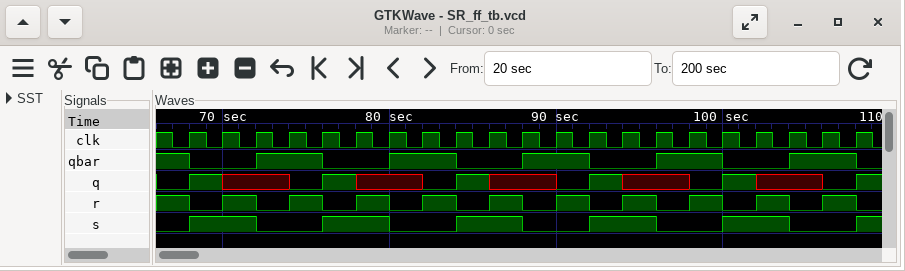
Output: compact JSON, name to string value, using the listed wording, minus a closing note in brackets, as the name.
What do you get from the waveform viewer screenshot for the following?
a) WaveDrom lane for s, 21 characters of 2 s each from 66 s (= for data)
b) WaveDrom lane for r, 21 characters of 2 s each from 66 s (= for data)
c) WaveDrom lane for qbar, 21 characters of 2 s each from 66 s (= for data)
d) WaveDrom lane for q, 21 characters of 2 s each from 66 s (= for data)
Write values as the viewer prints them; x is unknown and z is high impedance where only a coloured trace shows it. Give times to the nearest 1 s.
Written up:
{"WaveDrom lane for s, 21 characters of 2 s each from 66 s": "{name: 's', wave: '01.0.1.0.1.0.1.0.1.0.'}", "WaveDrom lane for r, 21 characters of 2 s each from 66 s": "{name: 'r', wave: '101010101010101010101'}", "WaveDrom lane for qbar, 21 characters of 2 s each from 66 s": "{name: 'qbar', wave: '10.1.0.1.0.1.0.1.0.1.'}", "WaveDrom lane for q, 21 characters of 2 s each from 66 s": "{name: 'q', wave: '01x.01x.01x.01x.01x.0'}"}
